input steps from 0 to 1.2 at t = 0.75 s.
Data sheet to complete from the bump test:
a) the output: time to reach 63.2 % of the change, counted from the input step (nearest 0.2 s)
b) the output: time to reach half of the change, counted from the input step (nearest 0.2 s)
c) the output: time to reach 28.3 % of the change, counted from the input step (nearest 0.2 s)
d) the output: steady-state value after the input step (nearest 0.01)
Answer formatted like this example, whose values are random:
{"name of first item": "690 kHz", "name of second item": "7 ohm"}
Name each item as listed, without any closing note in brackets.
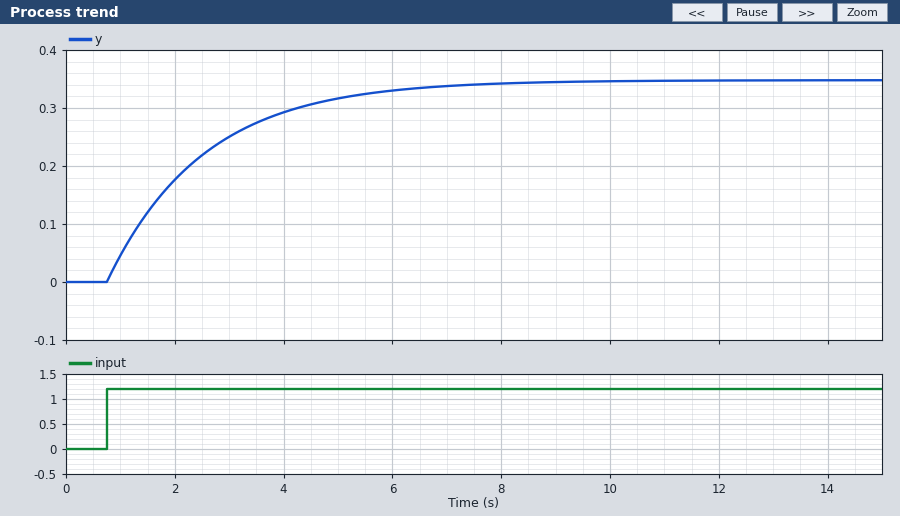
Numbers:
{"the output: time to reach 63.2 % of the change, counted from the input step": "1.8 s", "the output: time to reach half of the change, counted from the input step": "1.2 s", "the output: time to reach 28.3 % of the change, counted from the input step": "0.6 s", "the output: steady-state value after the input step": "0.35"}
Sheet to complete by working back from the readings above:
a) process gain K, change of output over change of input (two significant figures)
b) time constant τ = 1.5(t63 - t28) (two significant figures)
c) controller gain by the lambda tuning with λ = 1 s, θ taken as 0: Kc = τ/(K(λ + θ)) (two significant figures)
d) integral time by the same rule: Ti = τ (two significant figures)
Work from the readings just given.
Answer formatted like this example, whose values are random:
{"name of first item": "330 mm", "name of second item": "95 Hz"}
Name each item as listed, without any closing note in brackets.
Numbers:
{"process gain K, change of output over change of input": "0.29", "time constant τ = 1.5(t63 - t28)": "1.8 s", "controller gain by the lambda tuning with λ = 1 s, θ taken as 0: Kc = τ/(K(λ + θ))": "6.2", "integral time by the same rule: Ti = τ": "1.8 s"}
